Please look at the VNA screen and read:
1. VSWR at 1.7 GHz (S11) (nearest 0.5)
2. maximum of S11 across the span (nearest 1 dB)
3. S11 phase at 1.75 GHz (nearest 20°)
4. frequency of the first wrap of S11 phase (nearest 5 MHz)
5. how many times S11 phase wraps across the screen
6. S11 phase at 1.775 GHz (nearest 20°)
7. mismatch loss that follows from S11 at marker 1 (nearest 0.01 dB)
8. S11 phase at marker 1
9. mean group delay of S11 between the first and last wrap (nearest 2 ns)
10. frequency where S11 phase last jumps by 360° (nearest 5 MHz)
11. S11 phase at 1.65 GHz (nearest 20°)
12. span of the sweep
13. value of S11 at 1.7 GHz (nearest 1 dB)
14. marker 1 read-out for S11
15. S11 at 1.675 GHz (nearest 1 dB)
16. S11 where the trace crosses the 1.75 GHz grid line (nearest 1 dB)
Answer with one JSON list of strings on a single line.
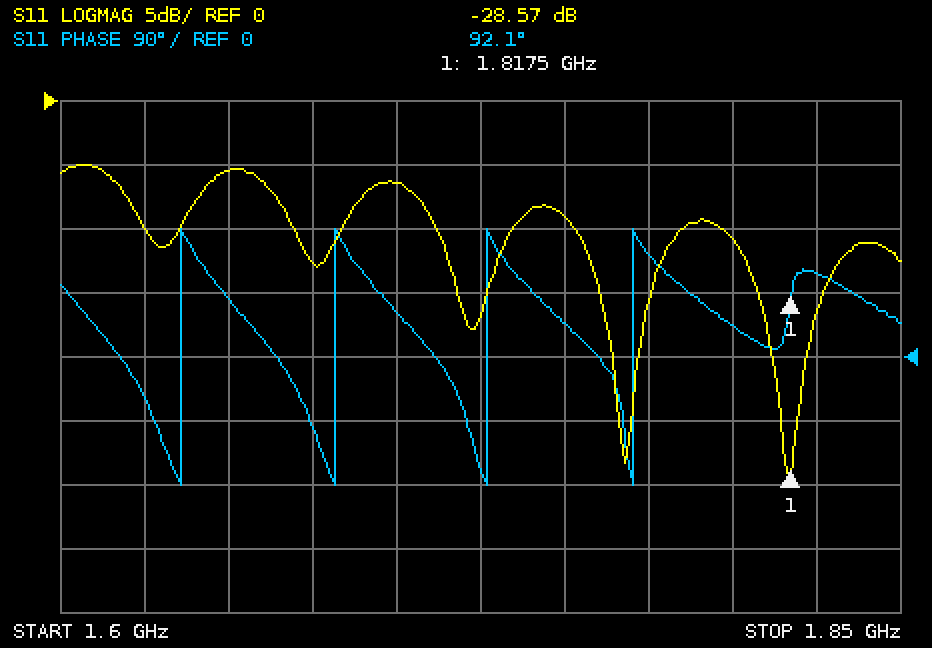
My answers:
["3.0", "-5 dB", "40°", "1.635 GHz", "4", "140°", "0.01 dB", "92.1°", "22 ns", "1.770 GHz", "80°", "250 MHz", "-6 dB", "-28.57 dB", "-13 dB", "-9 dB"]
